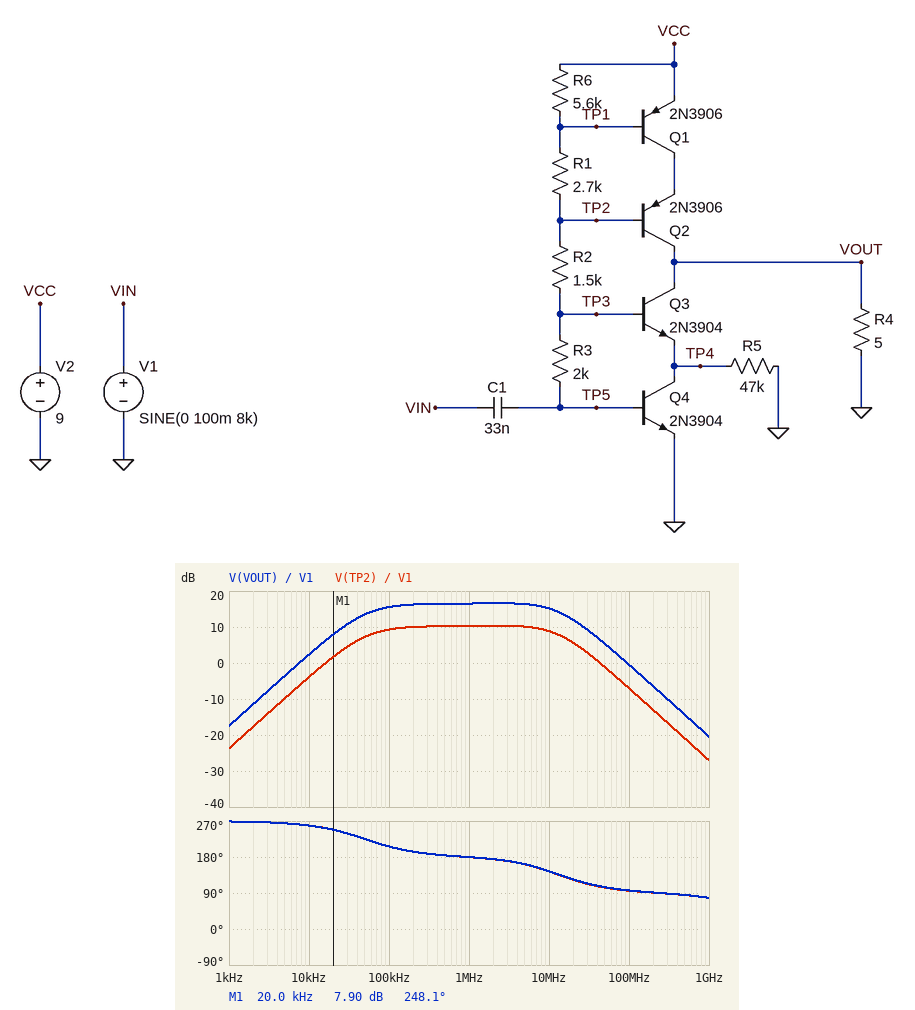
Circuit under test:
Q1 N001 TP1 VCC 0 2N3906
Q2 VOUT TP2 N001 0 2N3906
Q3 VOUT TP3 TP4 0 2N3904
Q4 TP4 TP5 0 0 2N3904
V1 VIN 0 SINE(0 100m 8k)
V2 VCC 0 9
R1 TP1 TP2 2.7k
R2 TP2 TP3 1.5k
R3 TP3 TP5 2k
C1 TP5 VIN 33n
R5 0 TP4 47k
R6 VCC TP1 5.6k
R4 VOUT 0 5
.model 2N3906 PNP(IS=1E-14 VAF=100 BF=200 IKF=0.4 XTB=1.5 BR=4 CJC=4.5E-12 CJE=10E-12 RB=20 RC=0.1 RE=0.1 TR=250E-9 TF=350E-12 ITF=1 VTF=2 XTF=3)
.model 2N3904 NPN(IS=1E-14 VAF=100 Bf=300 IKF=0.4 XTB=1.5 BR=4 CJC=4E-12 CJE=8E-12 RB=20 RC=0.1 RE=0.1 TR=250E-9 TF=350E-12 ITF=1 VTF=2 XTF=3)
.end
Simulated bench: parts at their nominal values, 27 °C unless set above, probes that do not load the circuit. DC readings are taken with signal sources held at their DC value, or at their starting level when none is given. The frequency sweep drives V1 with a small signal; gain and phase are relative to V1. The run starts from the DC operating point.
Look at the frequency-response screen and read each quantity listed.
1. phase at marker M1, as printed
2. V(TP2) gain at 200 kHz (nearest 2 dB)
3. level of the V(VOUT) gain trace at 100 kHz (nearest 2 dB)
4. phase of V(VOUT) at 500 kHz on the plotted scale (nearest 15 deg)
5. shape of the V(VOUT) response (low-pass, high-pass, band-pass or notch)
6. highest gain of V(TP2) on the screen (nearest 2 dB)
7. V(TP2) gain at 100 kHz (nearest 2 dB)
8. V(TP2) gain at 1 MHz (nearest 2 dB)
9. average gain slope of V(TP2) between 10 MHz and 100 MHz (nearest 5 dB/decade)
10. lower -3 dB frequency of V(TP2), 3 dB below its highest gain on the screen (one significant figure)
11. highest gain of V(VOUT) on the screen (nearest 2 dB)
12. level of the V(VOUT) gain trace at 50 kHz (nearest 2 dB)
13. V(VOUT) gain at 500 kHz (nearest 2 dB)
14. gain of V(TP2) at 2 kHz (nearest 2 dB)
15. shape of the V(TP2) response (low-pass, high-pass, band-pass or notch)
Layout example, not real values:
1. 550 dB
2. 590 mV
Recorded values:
1. 248.1 deg
2. 10 dB
3. 16 dB
4. 180 deg
5. band-pass
6. 10 dB
7. 10 dB
8. 10 dB
9. -15 dB/decade
10. 50 kHz
11. 16 dB
12. 14 dB
13. 16 dB
14. -18 dB
15. band-pass
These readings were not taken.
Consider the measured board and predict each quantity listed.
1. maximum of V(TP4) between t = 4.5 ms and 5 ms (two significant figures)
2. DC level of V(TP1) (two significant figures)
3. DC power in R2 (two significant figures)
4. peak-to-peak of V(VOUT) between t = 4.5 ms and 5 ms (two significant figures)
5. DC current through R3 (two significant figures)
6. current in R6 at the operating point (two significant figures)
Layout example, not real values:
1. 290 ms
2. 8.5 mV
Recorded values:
1. 560 mV
2. 8.2 V
3. 8.2 mW
4. 210 mV
5. 240 µA
6. 150 µA
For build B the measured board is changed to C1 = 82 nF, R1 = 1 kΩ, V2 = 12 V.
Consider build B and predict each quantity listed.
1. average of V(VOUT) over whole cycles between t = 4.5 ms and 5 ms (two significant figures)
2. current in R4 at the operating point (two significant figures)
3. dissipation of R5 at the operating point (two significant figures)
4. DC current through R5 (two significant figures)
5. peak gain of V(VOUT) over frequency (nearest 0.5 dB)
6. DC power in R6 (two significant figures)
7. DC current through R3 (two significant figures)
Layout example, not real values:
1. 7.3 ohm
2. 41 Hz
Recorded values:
1. 890 mV
2. 180 mA
3. 14 µW
4. 17 µA
5. 19.0 dB
6. 140 µW
7. 440 µA
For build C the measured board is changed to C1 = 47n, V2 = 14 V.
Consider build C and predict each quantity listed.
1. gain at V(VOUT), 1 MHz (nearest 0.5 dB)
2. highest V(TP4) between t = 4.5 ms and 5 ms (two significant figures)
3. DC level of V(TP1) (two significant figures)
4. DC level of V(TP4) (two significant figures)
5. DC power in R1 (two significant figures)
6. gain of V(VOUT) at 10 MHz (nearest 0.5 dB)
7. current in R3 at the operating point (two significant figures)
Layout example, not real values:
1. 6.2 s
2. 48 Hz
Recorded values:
1. 18.5 dB
2. 880 mV
3. 13 V
4. 720 mV
5. 12 mW
6. 16.0 dB
7. 390 µA
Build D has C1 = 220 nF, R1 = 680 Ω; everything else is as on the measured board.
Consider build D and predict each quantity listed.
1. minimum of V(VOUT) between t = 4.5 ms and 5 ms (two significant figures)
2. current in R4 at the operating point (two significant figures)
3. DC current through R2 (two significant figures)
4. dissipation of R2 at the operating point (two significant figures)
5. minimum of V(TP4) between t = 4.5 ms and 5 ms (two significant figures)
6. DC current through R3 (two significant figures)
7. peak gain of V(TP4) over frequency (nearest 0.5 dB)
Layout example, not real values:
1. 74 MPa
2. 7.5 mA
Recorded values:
1. 310 mV
2. 140 mA
3. 3.6 mA
4. 19 mW
5. 190 mV
6. 350 µA
7. 19.0 dB
